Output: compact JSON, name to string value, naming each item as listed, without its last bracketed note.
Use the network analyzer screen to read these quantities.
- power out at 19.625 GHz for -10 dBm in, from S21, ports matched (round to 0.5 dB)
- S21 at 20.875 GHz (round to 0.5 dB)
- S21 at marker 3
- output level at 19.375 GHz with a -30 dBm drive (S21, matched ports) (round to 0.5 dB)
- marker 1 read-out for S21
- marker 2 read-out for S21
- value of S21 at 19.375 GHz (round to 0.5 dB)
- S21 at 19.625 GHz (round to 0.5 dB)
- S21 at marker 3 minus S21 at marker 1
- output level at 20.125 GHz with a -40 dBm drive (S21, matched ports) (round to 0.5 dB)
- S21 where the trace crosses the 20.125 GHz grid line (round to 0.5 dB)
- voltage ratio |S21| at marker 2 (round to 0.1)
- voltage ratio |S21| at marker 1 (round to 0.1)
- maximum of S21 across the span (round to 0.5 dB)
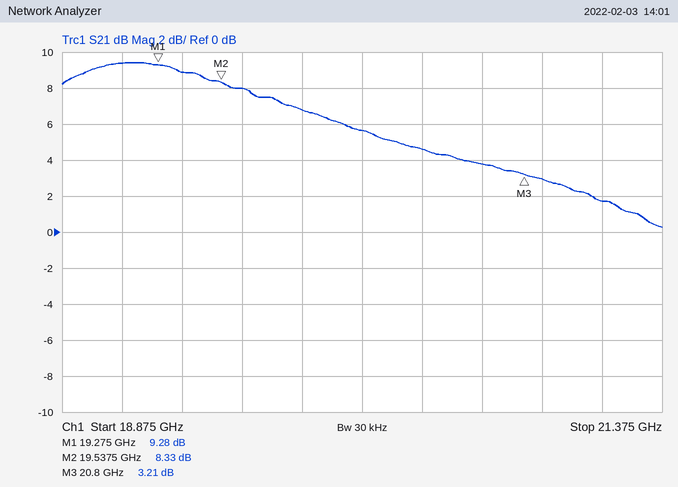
{"power out at 19.625 GHz for -10 dBm in, from S21, ports matched": "-2.0 dBm", "S21 at 20.875 GHz": "3.0 dB", "S21 at marker 3": "3.21 dB", "output level at 19.375 GHz with a -30 dBm drive (S21, matched ports)": "-21.0 dBm", "marker 1 read-out for S21": "9.28 dB", "marker 2 read-out for S21": "8.33 dB", "value of S21 at 19.375 GHz": "9.0 dB", "S21 at 19.625 GHz": "8.0 dB", "S21 at marker 3 minus S21 at marker 1": "-6.07 dB", "output level at 20.125 GHz with a -40 dBm drive (S21, matched ports)": "-34.5 dBm", "S21 where the trace crosses the 20.125 GHz grid line": "5.5 dB", "voltage ratio |S21| at marker 2": "2.6", "voltage ratio |S21| at marker 1": "2.9", "maximum of S21 across the span": "9.5 dB"}
